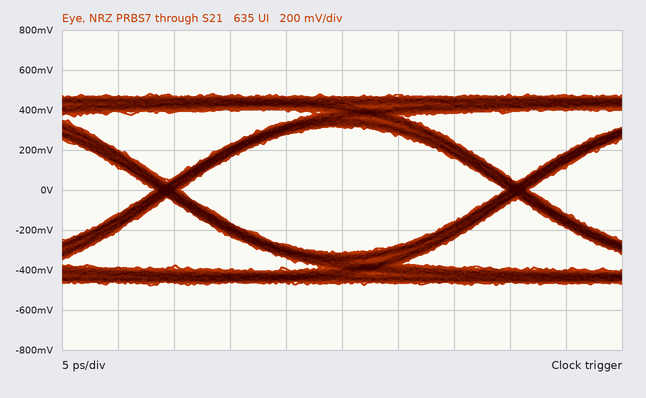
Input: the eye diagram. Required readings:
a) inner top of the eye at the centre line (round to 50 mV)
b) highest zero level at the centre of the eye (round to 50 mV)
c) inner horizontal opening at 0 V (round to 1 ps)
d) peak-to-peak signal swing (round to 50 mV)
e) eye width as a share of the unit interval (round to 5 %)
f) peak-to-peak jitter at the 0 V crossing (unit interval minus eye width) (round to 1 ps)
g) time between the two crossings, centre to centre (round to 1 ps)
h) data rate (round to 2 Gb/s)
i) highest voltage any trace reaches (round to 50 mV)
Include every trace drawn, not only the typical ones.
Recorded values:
300 mV
-300 mV
29 ps
950 mV
95 %
2 ps
31 ps
32 Gb/s
500 mV
